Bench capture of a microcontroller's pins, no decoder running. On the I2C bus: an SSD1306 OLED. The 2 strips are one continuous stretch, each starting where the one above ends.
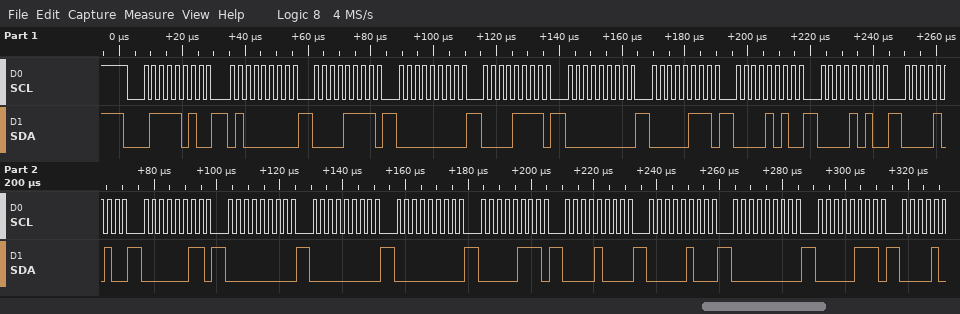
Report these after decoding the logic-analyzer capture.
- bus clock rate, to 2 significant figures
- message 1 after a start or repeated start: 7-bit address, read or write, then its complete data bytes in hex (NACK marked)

400 kHz
0x3D write: 40 0F 00 0F 00 07 0A 0A 0A 03 00 00 00 07 08 04 00 07
